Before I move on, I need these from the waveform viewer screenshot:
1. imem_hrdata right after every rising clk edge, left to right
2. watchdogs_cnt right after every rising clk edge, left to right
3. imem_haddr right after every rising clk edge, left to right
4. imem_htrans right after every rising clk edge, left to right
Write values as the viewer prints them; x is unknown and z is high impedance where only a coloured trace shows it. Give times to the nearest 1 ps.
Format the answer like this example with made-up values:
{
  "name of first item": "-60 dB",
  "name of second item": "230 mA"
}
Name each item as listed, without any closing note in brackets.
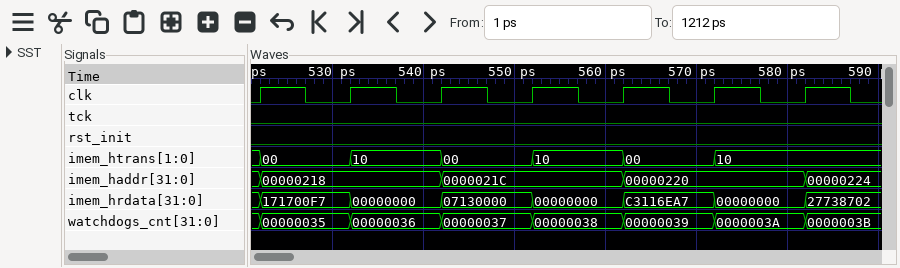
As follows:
{
  "imem_hrdata right after every rising clk edge, left to right": "171700F7, 00000000, 07130000, 00000000, C3116EA7, 00000000, 27738702",
  "watchdogs_cnt right after every rising clk edge, left to right": "00000035, 00000036, 00000037, 00000038, 00000039, 0000003A, 0000003B",
  "imem_haddr right after every rising clk edge, left to right": "00000218, 00000218, 0000021C, 0000021C, 00000220, 00000220, 00000224",
  "imem_htrans right after every rising clk edge, left to right": "00, 10, 00, 10, 00, 10, 10"
}
